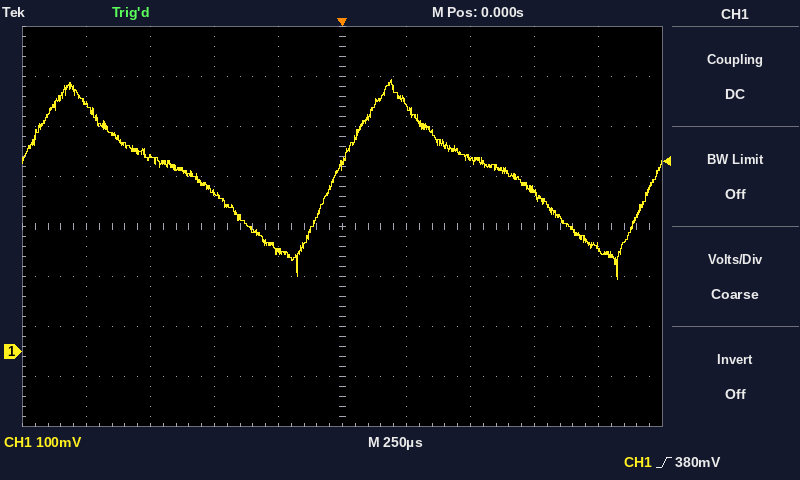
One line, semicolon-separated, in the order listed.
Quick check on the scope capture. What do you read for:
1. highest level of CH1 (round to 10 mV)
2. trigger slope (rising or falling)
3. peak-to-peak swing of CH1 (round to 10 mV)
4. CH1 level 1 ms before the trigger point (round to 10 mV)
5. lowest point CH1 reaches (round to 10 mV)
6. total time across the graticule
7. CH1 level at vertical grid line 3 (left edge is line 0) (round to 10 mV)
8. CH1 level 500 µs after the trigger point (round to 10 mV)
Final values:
540 mV; rising; 400 mV; 500 mV; 140 mV; 2.5 ms; 320 mV; 390 mV
